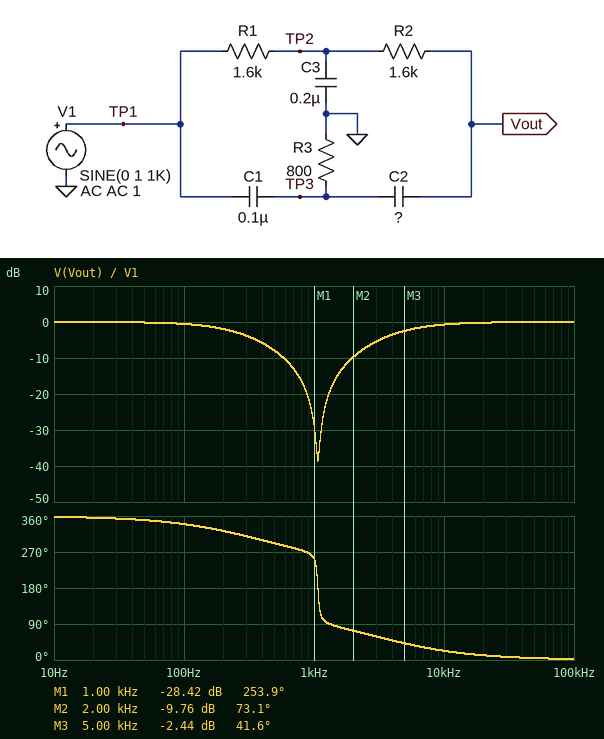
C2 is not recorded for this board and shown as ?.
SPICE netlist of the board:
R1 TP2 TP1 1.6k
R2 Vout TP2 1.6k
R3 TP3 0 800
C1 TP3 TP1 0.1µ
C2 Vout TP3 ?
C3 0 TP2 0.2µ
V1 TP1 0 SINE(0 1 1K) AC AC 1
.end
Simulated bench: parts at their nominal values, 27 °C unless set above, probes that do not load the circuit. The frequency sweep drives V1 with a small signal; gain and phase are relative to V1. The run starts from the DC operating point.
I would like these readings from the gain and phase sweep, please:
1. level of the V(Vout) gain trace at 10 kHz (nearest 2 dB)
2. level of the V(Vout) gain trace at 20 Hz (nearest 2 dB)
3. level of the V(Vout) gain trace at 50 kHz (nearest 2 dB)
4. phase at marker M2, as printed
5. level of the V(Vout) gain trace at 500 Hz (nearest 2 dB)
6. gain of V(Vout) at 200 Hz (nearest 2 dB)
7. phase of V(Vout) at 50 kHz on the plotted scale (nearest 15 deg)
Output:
0 dB
0 dB
0 dB
73.1 deg
-8 dB
-2 dB
0 deg
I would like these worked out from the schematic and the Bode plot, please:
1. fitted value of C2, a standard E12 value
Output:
82 nF
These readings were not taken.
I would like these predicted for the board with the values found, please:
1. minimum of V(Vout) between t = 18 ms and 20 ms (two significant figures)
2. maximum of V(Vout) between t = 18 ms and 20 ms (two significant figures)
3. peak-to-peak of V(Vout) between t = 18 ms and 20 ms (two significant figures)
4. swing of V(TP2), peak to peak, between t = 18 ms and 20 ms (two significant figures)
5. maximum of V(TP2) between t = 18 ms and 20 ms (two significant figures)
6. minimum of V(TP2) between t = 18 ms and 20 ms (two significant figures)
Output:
-38 mV
38 mV
76 mV
700 mV
350 mV
-350 mV
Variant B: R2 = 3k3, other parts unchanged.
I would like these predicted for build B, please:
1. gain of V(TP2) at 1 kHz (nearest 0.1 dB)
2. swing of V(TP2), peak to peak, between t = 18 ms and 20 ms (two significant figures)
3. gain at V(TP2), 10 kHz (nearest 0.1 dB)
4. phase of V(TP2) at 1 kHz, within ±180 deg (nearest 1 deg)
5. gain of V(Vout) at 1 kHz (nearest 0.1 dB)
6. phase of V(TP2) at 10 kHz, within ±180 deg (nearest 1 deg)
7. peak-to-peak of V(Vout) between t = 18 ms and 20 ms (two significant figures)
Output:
-8.1 dB
790 mV
-22.9 dB
-50 deg
-17.9 dB
-80 deg
250 mV
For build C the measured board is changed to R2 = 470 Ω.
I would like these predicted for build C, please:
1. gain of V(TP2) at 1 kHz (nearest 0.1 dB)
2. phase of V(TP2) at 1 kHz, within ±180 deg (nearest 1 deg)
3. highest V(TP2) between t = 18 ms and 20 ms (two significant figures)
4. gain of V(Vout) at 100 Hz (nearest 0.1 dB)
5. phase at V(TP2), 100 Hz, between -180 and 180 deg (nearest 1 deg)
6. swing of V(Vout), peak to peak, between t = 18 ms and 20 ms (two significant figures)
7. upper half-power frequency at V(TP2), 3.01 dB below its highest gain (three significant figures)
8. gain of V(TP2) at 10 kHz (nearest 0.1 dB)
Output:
-10.5 dB
-48 deg
300 mV
-0.4 dB
-16 deg
390 mV
313 Hz
-16.3 dB
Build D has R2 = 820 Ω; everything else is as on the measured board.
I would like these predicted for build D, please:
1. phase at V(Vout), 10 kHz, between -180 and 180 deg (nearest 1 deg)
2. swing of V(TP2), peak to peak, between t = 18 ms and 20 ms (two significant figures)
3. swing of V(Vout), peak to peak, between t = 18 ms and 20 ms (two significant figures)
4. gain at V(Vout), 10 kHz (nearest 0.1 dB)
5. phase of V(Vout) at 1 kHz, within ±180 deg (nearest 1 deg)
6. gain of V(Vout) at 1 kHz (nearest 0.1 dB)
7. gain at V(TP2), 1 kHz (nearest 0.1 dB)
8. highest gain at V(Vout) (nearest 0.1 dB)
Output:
32 deg
630 mV
280 mV
-1.6 dB
-69 deg
-17.1 dB
-10.0 dB
0 dB
